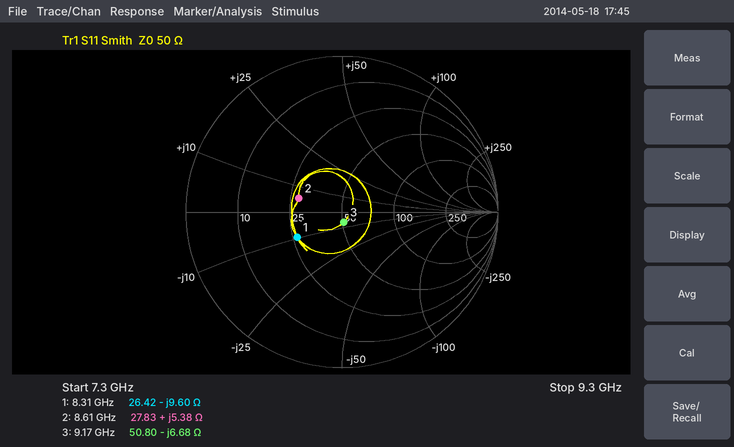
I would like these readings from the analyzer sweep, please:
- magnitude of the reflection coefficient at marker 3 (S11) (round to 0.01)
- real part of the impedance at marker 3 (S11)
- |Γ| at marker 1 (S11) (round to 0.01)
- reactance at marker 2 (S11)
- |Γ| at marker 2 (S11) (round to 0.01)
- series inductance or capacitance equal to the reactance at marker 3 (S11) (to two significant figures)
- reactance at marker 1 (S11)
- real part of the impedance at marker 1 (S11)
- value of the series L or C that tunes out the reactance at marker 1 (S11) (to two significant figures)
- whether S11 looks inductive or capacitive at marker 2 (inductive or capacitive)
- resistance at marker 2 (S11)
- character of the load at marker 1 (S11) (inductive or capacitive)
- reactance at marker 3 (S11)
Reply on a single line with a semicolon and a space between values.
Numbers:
0.07; 50.80 Ω; 0.33; +5.38 Ω; 0.29; 2.6 pF; -9.60 Ω; 26.42 Ω; 180 pH; inductive; 27.83 Ω; capacitive; -6.68 Ω
